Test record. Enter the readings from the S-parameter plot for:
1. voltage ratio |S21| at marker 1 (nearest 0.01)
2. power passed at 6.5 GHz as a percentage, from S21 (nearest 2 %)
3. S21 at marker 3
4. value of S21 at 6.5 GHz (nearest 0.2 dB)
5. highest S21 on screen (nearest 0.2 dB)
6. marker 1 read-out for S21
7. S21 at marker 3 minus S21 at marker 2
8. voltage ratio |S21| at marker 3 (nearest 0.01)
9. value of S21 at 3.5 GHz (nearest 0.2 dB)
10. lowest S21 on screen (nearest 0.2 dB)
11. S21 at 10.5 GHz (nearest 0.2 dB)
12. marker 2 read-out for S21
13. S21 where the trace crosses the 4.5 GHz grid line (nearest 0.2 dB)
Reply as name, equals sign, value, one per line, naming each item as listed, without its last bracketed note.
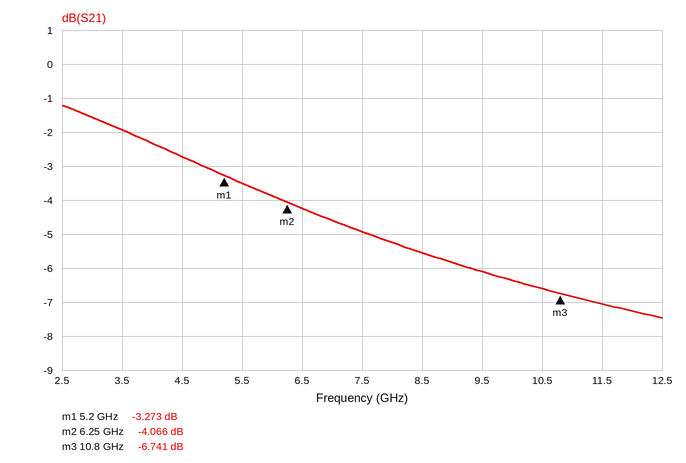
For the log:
voltage ratio |S21| at marker 1 = 0.69
power passed at 6.5 GHz as a percentage, from S21 = 38 %
S21 at marker 3 = -6.741 dB
value of S21 at 6.5 GHz = -4.2 dB
highest S21 on screen = -1.2 dB
marker 1 read-out for S21 = -3.273 dB
S21 at marker 3 minus S21 at marker 2 = -2.675 dB
voltage ratio |S21| at marker 3 = 0.46
value of S21 at 3.5 GHz = -2.0 dB
lowest S21 on screen = -7.4 dB
S21 at 10.5 GHz = -6.6 dB
marker 2 read-out for S21 = -4.066 dB
S21 where the trace crosses the 4.5 GHz grid line = -2.8 dB
